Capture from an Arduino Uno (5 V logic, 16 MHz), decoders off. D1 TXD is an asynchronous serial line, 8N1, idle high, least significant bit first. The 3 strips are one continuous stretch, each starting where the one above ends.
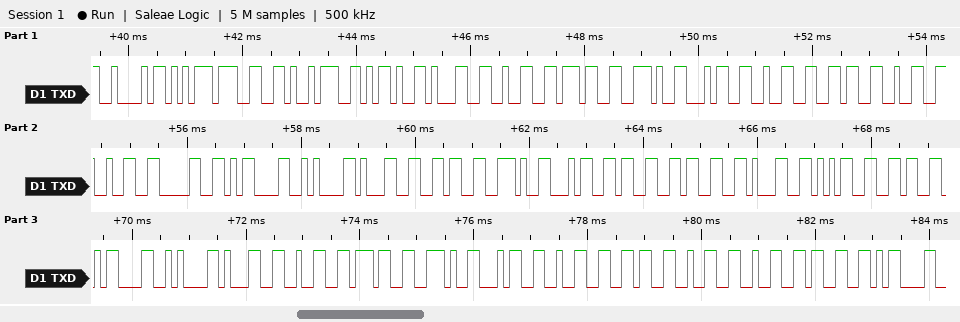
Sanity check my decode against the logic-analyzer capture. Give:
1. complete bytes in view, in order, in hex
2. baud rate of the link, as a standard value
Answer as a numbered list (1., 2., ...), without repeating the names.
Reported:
1. 42 75 66 3A 2D 31 32 37 2E 34 32 36 32 32 30 0D 0A 31 36 2E 34 33 33 31 35 36 0D 0A 31 32 37 2E 34 32 36 32 32 33 0D
2. 9600 baud
